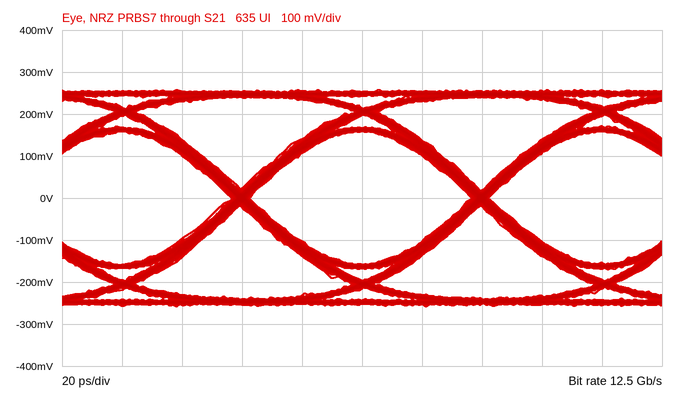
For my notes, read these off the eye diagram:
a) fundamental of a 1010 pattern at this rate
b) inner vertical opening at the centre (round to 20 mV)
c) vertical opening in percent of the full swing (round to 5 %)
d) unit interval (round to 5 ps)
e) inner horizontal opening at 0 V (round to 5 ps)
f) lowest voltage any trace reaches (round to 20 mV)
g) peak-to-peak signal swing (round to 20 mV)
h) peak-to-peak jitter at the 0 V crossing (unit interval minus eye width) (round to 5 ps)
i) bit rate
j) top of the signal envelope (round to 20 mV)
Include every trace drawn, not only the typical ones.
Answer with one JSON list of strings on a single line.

["6.25 GHz", "320 mV", "60 %", "80 ps", "75 ps", "-260 mV", "520 mV", "5 ps", "12.5 Gb/s", "260 mV"]
